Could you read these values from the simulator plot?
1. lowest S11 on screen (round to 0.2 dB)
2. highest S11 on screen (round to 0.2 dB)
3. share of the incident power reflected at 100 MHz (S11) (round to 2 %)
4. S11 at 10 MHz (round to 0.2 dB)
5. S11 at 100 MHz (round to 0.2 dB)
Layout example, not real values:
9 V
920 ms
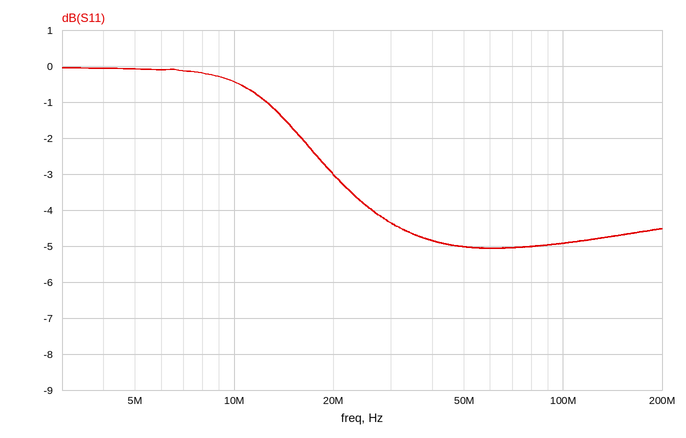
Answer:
-5.0 dB
0.0 dB
32 %
-0.4 dB
-5.0 dB
